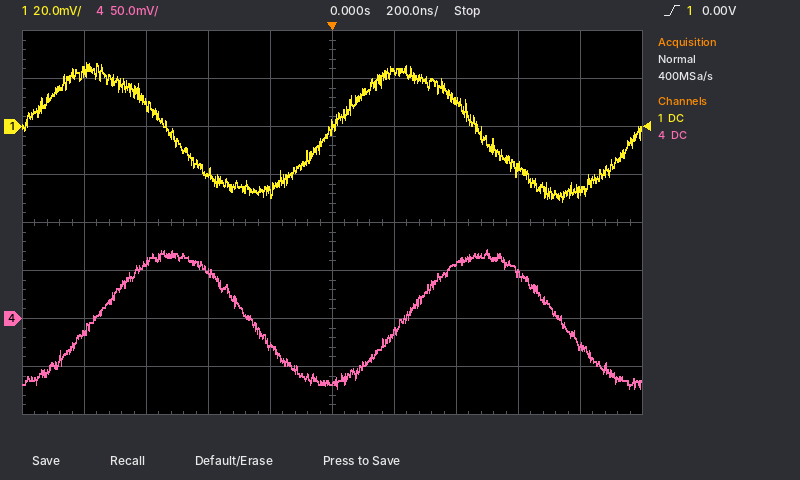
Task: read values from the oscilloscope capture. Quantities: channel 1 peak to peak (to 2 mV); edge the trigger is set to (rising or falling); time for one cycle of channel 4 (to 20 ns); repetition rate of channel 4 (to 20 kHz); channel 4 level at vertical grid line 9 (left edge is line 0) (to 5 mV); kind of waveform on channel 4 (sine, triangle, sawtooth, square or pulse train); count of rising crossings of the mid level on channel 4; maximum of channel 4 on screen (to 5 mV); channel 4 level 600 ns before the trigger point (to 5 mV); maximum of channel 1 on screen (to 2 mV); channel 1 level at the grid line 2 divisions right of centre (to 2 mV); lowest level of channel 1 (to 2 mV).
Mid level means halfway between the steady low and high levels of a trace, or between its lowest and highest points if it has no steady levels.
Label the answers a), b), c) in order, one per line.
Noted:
a) 58 mV
b) rising
c) 1.00 µs
d) 1.00 MHz
e) -30 mV
f) sine
g) 2
h) 70 mV
i) 60 mV
j) 26 mV
k) 10 mV
l) -32 mV
